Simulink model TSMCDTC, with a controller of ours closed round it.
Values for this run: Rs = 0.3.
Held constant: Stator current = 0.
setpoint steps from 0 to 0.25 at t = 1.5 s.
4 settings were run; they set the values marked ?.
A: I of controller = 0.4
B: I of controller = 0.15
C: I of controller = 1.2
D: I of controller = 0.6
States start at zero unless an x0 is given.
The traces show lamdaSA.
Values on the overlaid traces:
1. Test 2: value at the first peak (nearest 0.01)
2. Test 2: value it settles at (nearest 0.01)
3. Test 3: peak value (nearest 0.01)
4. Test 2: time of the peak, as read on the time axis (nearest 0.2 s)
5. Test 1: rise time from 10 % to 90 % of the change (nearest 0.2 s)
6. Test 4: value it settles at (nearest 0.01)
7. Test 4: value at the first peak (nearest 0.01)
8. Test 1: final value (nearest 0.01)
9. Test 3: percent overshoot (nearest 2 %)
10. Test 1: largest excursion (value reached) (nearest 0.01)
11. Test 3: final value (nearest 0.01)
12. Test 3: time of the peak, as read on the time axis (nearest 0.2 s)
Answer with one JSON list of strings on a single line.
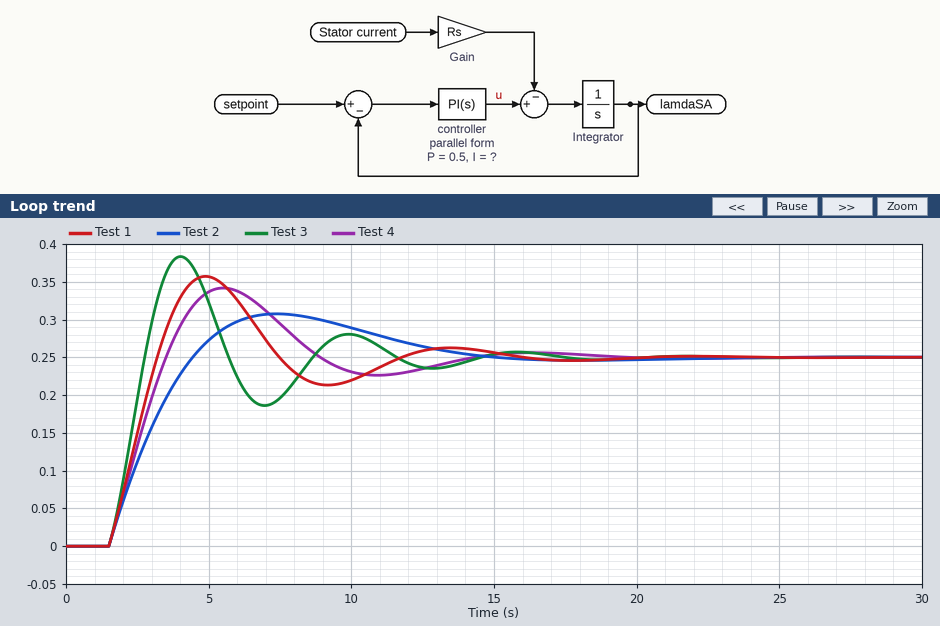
["0.31", "0.25", "0.38", "7.4 s", "1.4 s", "0.25", "0.34", "0.25", "54 %", "0.36", "0.25", "4.0 s"]
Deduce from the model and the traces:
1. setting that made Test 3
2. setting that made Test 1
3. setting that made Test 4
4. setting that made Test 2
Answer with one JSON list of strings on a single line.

["C", "D", "A", "B"]
